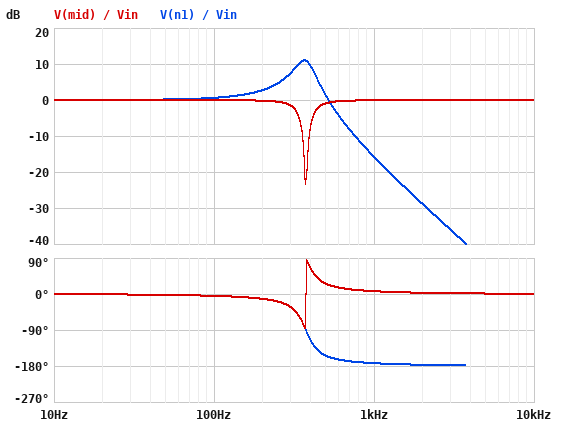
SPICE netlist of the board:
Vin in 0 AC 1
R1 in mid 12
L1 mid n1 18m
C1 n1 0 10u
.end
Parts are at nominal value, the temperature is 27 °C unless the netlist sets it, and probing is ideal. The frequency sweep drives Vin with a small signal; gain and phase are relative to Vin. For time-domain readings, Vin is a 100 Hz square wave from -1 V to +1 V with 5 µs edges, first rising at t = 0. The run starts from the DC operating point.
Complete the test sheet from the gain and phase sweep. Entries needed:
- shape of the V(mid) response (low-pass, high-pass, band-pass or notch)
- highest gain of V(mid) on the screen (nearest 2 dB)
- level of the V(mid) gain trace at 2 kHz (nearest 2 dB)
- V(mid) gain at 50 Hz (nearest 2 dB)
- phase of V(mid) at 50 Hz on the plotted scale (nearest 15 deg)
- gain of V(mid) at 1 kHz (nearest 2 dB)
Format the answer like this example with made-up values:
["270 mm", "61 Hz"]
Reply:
["notch", "0 dB", "0 dB", "0 dB", "0 deg", "0 dB"]
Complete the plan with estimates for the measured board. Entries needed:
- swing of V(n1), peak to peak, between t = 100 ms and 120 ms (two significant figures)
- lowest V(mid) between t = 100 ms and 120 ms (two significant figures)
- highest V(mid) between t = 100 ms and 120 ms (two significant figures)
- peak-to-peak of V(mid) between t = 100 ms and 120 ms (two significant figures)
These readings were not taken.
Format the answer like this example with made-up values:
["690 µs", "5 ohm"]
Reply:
["4.3 V", "-1.3 V", "1.3 V", "2.5 V"]
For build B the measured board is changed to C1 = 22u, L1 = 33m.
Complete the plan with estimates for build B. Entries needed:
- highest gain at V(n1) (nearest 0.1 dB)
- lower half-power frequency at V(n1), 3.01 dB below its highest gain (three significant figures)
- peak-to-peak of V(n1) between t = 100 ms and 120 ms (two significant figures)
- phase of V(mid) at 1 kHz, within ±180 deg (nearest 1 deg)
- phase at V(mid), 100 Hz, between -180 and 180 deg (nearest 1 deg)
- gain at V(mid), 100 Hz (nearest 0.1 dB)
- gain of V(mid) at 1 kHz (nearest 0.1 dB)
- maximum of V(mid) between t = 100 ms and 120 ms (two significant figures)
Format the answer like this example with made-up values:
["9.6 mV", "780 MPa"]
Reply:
["10.3 dB", "150 Hz", "3.8 V", "3 deg", "-13 deg", "-0.2 dB", "0 dB", "1.2 V"]
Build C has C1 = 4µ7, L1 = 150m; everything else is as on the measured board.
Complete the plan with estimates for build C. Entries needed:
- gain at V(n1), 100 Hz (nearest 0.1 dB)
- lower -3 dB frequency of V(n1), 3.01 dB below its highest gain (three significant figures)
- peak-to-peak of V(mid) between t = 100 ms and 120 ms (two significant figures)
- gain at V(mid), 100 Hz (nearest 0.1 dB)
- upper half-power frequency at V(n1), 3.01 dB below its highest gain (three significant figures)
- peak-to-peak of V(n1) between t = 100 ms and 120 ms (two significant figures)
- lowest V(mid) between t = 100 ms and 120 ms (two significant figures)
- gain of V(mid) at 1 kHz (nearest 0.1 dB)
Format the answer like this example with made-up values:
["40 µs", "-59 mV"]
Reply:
["2.8 dB", "183 Hz", "2.1 V", "0 dB", "196 Hz", "4.0 V", "-1.1 V", "0 dB"]
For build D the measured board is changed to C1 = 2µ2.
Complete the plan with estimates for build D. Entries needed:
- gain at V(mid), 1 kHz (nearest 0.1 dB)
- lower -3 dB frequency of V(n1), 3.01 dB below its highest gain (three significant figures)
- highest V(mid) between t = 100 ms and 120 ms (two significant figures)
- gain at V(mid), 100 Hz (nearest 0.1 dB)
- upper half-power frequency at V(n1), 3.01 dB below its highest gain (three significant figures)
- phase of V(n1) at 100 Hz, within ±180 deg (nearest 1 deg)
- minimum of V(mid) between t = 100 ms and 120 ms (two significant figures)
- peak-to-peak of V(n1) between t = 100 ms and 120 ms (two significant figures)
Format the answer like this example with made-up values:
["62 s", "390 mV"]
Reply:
["-0.4 dB", "741 Hz", "1.2 V", "0 dB", "848 Hz", "-1 deg", "-1.2 V", "4.7 V"]
